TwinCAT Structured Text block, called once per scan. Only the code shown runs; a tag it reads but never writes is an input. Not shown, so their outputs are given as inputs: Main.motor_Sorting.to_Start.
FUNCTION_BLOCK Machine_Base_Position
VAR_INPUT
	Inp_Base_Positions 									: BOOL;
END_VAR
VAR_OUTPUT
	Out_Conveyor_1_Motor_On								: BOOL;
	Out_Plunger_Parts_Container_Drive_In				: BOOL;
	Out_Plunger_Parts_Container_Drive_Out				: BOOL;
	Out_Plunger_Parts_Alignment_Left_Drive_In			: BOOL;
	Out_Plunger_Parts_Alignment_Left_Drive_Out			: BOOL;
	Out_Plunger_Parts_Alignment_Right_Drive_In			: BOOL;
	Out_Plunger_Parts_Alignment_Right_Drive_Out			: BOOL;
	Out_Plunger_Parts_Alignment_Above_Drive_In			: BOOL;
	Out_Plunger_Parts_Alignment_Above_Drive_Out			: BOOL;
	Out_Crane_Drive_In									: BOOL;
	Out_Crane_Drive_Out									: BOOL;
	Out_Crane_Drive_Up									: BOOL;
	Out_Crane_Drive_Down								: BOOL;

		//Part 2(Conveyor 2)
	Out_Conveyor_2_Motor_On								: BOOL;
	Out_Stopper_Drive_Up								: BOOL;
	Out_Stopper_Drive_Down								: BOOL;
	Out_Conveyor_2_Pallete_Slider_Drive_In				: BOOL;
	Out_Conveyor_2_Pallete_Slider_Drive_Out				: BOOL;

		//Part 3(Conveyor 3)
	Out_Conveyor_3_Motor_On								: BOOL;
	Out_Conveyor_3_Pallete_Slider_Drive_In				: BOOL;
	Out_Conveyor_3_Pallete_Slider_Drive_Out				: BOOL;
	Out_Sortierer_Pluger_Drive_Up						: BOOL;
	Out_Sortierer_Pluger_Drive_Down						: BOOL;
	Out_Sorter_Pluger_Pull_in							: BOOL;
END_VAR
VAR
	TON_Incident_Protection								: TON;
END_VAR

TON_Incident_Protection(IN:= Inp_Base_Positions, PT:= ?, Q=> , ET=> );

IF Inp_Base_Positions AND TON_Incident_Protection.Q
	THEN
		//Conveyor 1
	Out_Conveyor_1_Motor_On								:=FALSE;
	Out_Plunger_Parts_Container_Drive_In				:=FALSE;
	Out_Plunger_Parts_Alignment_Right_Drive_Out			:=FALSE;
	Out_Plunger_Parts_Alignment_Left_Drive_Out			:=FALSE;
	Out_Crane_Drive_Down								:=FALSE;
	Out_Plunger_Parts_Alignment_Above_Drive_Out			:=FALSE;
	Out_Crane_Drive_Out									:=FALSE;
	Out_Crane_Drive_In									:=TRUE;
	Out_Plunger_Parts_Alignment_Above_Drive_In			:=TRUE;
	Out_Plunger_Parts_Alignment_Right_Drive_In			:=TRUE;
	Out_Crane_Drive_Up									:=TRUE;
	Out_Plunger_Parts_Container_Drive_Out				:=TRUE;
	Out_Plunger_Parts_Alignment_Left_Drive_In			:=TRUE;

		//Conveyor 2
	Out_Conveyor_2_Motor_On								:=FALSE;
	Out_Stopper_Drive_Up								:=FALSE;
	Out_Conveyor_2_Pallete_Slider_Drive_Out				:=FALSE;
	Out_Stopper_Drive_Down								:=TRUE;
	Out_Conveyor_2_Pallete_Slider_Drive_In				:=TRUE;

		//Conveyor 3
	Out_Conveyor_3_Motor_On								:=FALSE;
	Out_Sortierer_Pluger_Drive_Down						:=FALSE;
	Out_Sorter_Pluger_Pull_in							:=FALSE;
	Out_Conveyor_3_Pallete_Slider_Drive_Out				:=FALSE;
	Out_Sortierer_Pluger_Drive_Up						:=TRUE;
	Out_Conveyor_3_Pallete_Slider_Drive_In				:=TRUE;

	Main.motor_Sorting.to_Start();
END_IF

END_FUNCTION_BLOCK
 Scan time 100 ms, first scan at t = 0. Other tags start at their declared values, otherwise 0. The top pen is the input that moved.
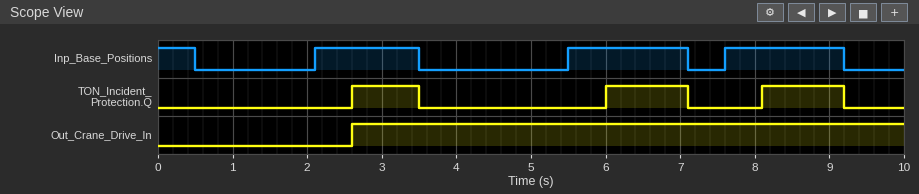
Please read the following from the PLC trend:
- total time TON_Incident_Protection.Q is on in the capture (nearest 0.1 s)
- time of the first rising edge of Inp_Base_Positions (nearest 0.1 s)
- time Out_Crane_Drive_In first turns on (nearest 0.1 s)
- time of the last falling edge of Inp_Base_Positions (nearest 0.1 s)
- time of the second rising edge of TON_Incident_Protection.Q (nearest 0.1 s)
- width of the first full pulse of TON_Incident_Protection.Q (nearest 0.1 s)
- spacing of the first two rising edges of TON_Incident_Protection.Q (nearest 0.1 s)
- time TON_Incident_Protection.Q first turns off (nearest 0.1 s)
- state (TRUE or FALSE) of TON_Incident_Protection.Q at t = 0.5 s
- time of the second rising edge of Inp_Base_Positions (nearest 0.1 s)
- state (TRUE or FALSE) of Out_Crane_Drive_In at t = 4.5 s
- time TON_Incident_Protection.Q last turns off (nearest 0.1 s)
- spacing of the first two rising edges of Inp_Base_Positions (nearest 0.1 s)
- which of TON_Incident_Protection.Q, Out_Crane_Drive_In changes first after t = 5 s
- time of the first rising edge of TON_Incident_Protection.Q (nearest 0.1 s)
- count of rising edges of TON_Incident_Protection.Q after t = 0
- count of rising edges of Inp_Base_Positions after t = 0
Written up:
3.1 s
2.1 s
2.6 s
9.2 s
6.0 s
0.9 s
3.4 s
3.5 s
FALSE
5.5 s
TRUE
9.2 s
3.4 s
TON_Incident_Protection.Q
2.6 s
3
3
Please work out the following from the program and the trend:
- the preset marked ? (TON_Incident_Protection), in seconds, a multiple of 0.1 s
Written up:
0.5 s
